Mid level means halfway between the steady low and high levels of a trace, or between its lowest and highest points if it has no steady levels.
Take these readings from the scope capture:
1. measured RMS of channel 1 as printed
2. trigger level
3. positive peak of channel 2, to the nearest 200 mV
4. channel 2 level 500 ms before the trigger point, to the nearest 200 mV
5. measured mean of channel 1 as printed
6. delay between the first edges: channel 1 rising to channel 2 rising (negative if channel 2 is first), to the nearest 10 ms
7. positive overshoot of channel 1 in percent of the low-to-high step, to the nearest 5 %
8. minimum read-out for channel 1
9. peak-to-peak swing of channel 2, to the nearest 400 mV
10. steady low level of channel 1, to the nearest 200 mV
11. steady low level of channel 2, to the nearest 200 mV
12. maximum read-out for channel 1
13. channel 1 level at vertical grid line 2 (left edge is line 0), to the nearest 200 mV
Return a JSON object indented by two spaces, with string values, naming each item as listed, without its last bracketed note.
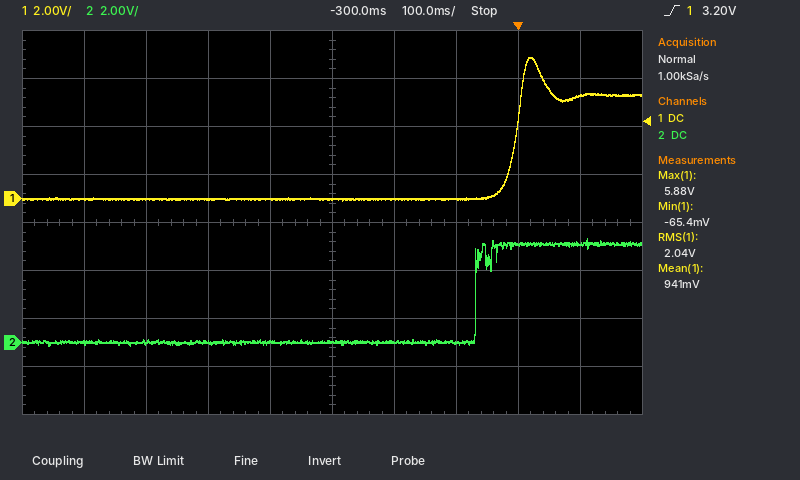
{
  "measured RMS of channel 1 as printed": "2.04 V",
  "trigger level": "3.20 V",
  "positive peak of channel 2, to the nearest 200 mV": "4.4 V",
  "channel 2 level 500 ms before the trigger point, to the nearest 200 mV": "0.0 V",
  "measured mean of channel 1 as printed": "941 mV",
  "delay between the first edges: channel 1 rising to channel 2 rising (negative if channel 2 is first), to the nearest 10 ms": "-60 ms",
  "positive overshoot of channel 1 in percent of the low-to-high step, to the nearest 5 %": "35 %",
  "minimum read-out for channel 1": "-65.4 mV",
  "peak-to-peak swing of channel 2, to the nearest 400 mV": "4.4 V",
  "steady low level of channel 1, to the nearest 200 mV": "0.0 V",
  "steady low level of channel 2, to the nearest 200 mV": "0.0 V",
  "maximum read-out for channel 1": "5.88 V",
  "channel 1 level at vertical grid line 2 (left edge is line 0), to the nearest 200 mV": "0.0 V"
}
